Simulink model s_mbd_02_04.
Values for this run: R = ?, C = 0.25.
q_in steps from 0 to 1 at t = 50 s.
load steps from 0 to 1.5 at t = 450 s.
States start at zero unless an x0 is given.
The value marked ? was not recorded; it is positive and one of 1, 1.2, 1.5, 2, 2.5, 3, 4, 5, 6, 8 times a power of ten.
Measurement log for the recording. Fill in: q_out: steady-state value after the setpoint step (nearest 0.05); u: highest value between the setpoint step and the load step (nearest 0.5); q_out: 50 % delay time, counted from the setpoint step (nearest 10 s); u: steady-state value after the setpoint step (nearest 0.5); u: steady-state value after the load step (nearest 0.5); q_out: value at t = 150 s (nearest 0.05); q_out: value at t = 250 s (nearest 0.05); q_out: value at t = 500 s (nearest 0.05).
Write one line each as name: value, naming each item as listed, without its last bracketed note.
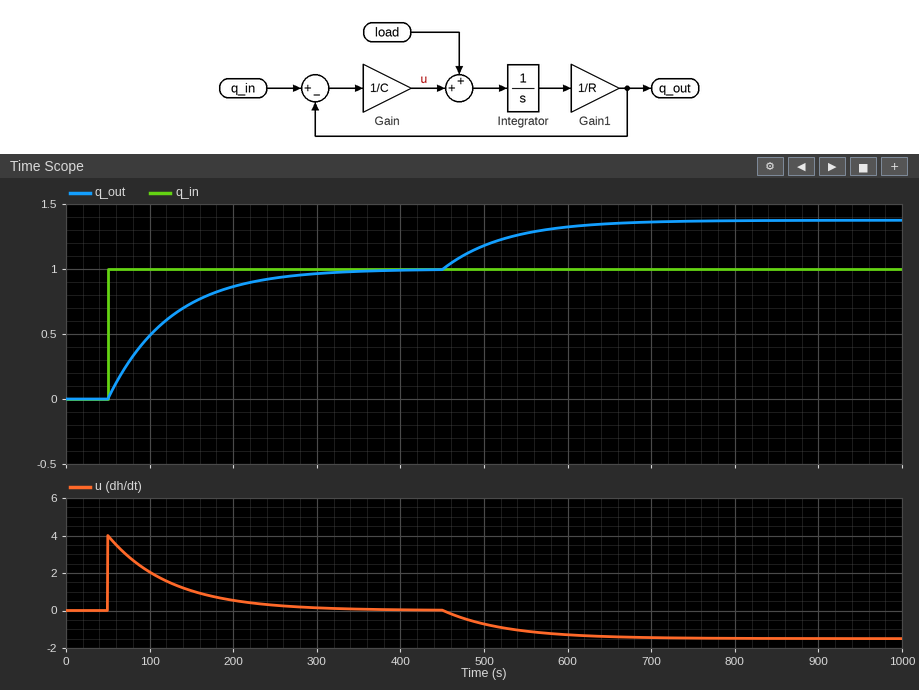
q_out: steady-state value after the setpoint step: 1.00
u: highest value between the setpoint step and the load step: 4.0
q_out: 50 % delay time, counted from the setpoint step: 50 s
u: steady-state value after the setpoint step: 0.0
u: steady-state value after the load step: -1.5
q_out: value at t = 150 s: 0.75
q_out: value at t = 250 s: 0.95
q_out: value at t = 500 s: 1.20
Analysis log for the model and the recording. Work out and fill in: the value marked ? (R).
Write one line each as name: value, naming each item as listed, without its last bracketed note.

the value marked ?: 300
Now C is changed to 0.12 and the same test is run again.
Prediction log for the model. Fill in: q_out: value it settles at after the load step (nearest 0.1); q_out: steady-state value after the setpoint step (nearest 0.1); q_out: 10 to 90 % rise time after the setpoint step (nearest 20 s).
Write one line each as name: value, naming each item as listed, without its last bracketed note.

q_out: value it settles at after the load step: 1.2
q_out: steady-state value after the setpoint step: 1.0
q_out: 10 to 90 % rise time after the setpoint step: 80 s
